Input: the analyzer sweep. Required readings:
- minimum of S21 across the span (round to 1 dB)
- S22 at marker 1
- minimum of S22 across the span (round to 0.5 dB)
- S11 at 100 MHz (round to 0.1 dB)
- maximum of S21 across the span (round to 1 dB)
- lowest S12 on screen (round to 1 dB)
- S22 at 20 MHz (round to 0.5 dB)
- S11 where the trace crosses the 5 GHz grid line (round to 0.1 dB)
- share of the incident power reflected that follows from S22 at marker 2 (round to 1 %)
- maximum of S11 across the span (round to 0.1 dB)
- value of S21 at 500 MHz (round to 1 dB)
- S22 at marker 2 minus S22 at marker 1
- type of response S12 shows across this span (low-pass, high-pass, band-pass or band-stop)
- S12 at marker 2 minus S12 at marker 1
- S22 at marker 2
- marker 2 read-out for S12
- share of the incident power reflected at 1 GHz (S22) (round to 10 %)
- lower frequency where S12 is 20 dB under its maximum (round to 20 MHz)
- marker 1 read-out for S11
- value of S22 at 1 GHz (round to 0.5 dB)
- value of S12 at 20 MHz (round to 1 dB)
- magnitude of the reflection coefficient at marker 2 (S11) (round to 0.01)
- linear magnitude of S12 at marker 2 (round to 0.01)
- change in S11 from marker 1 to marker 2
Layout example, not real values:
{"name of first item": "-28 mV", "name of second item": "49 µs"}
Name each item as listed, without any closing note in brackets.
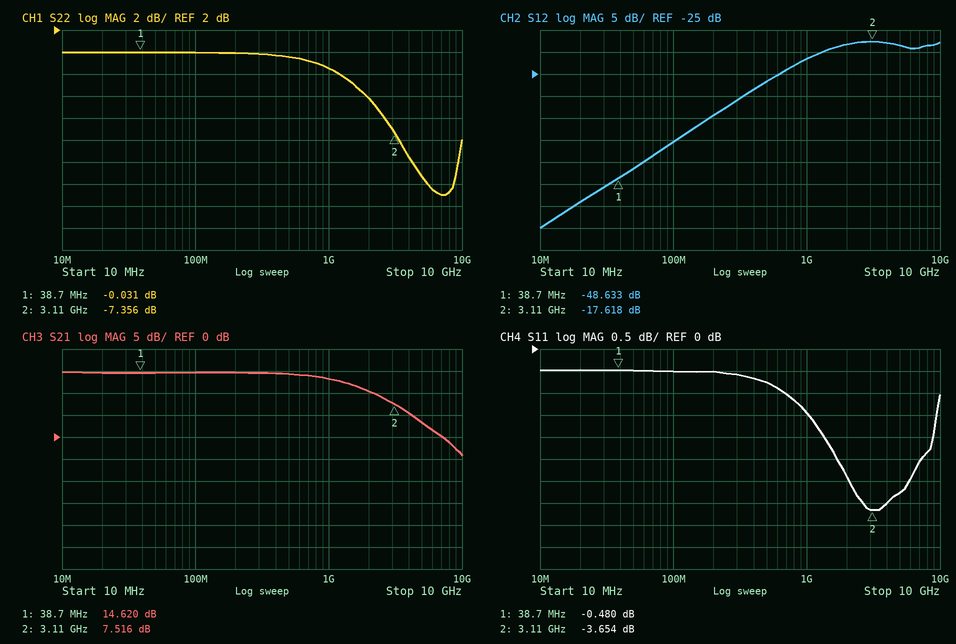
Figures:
{"minimum of S21 across the span": "-4 dB", "S22 at marker 1": "-0.031 dB", "minimum of S22 across the span": "-13.0 dB", "S11 at 100 MHz": "-0.5 dB", "maximum of S21 across the span": "15 dB", "lowest S12 on screen": "-60 dB", "S22 at 20 MHz": "0.0 dB", "S11 where the trace crosses the 5 GHz grid line": "-3.3 dB", "share of the incident power reflected that follows from S22 at marker 2": "18 %", "maximum of S11 across the span": "-0.5 dB", "value of S21 at 500 MHz": "14 dB", "S22 at marker 2 minus S22 at marker 1": "-7.325 dB", "type of response S12 shows across this span": "high-pass", "S12 at marker 2 minus S12 at marker 1": "31.015 dB", "S22 at marker 2": "-7.356 dB", "marker 2 read-out for S12": "-17.618 dB", "share of the incident power reflected at 1 GHz (S22)": "70 %", "lower frequency where S12 is 20 dB under its maximum": "140 MHz", "marker 1 read-out for S11": "-0.480 dB", "value of S22 at 1 GHz": "-1.5 dB", "value of S12 at 20 MHz": "-54 dB", "magnitude of the reflection coefficient at marker 2 (S11)": "0.66", "linear magnitude of S12 at marker 2": "0.13", "change in S11 from marker 1 to marker 2": "-3.174 dB"}
